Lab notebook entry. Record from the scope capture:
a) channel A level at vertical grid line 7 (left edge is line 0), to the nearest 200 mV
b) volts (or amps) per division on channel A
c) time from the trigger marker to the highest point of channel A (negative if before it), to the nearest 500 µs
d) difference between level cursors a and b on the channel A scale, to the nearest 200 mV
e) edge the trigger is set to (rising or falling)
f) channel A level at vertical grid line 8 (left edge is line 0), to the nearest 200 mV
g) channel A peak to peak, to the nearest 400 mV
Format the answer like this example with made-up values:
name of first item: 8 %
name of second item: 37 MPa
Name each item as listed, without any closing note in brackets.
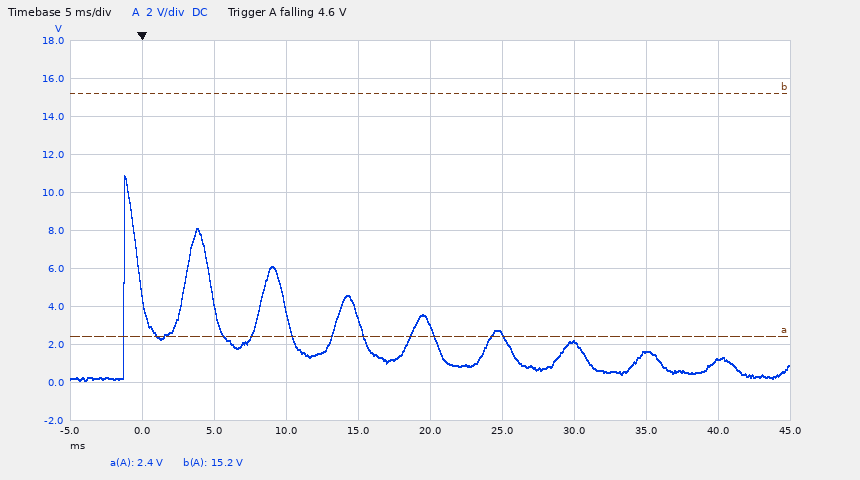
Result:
channel A level at vertical grid line 7 (left edge is line 0), to the nearest 200 mV: 2.2 V
volts (or amps) per division on channel A: 2 V
time from the trigger marker to the highest point of channel A (negative if before it), to the nearest 500 µs: -1.0 ms
difference between level cursors a and b on the channel A scale, to the nearest 200 mV: 12.8 V
edge the trigger is set to: falling
channel A level at vertical grid line 8 (left edge is line 0), to the nearest 200 mV: 1.6 V
channel A peak to peak, to the nearest 400 mV: 10.8 V
